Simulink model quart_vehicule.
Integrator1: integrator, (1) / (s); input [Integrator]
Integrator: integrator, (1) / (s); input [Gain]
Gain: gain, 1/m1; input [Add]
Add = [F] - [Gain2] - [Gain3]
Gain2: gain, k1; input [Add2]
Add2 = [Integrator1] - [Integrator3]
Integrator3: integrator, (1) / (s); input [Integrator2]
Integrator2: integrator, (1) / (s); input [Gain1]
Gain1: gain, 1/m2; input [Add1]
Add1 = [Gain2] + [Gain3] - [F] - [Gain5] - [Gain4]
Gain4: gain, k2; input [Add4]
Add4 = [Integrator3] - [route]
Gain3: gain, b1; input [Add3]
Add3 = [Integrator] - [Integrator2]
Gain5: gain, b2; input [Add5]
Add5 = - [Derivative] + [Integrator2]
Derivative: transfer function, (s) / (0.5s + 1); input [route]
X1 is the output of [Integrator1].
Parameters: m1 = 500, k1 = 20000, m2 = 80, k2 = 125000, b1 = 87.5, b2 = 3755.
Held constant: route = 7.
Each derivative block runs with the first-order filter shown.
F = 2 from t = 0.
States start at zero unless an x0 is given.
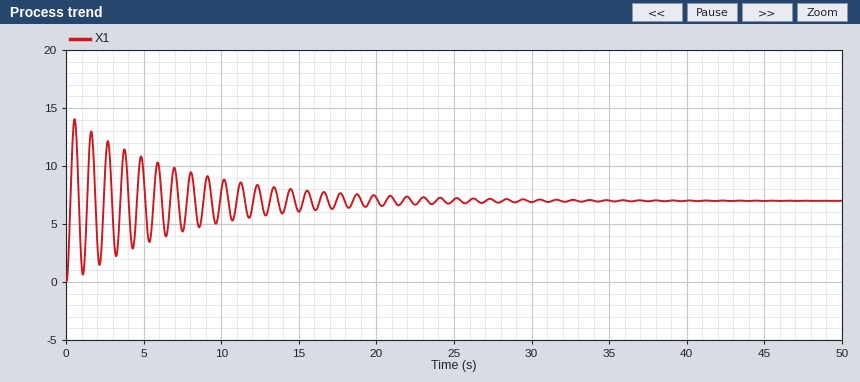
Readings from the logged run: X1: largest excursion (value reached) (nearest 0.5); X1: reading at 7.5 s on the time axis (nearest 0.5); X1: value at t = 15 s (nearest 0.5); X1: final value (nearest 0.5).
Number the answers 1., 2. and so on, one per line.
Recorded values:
1. 14.0
2. 4.5
3. 6.0
4. 7.0
